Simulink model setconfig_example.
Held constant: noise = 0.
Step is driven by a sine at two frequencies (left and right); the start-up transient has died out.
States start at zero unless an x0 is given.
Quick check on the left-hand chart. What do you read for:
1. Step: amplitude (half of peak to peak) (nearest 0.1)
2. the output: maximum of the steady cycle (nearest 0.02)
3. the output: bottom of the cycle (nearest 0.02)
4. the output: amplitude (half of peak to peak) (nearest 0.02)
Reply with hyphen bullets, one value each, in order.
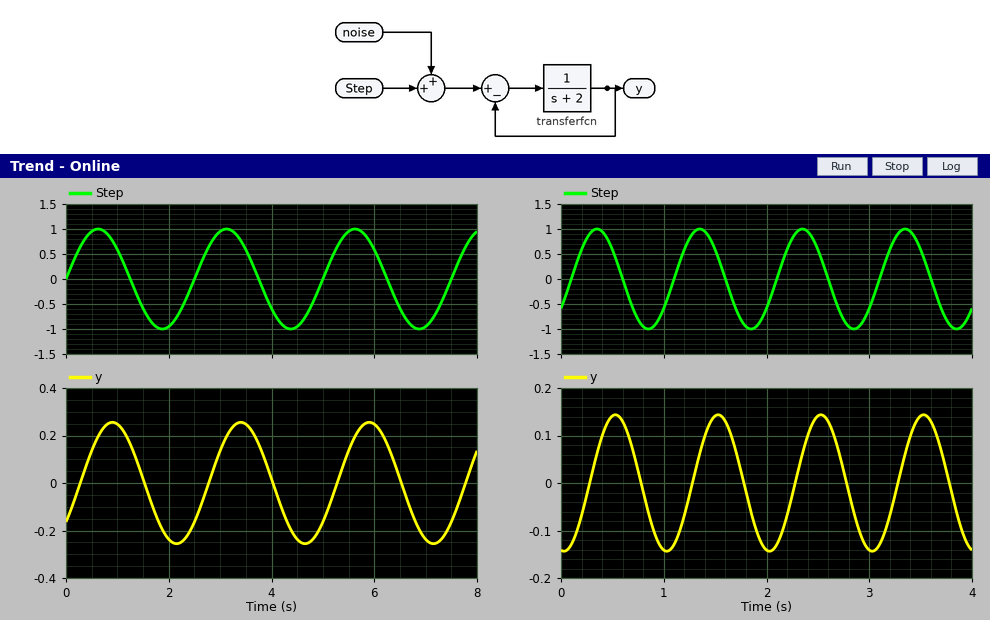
- 1.0
- 0.26
- -0.26
- 0.26
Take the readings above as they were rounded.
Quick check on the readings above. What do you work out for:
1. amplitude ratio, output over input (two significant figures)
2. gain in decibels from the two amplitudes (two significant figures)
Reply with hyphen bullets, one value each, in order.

- 0.26
- -12 dB
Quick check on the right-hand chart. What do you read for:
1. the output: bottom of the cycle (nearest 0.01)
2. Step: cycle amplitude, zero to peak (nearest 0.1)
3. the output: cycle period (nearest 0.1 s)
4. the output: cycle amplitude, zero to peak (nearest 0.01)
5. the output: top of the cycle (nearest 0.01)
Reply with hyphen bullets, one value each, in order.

- -0.14
- 1.0
- 1.0 s
- 0.14
- 0.14
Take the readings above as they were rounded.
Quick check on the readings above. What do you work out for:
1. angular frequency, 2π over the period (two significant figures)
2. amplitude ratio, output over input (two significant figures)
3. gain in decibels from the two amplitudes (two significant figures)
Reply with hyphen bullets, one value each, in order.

- 6.3 rad/s
- 0.14
- -17 dB
